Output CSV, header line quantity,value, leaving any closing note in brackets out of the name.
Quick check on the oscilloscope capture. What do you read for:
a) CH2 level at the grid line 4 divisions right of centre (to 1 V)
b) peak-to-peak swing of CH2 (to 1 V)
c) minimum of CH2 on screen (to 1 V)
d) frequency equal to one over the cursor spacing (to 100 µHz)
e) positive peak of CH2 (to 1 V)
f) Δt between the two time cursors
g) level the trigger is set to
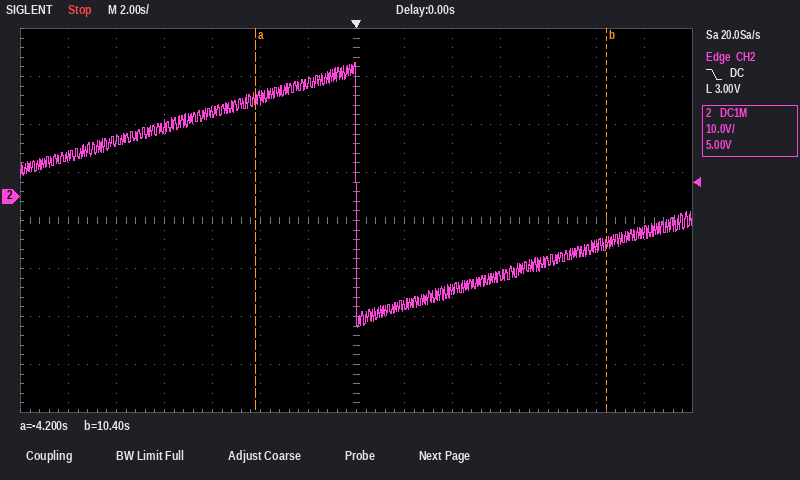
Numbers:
quantity,value
CH2 level at the grid line 4 divisions right of centre,-13 V
peak-to-peak swing of CH2,55 V
minimum of CH2 on screen,-27 V
frequency equal to one over the cursor spacing,68.5 mHz
positive peak of CH2,28 V
Δt between the two time cursors,14.6 s
level the trigger is set to,3.00 V
